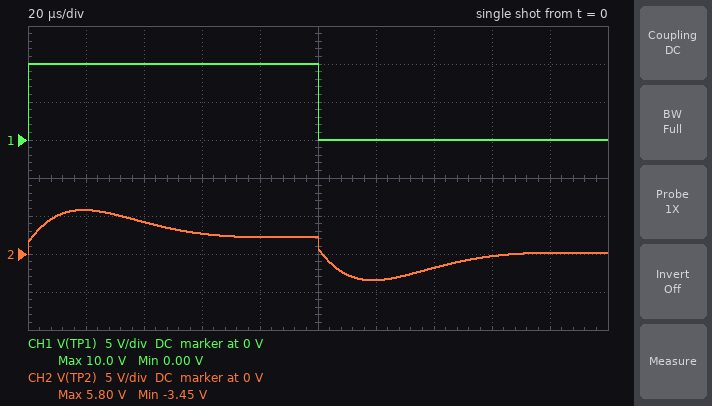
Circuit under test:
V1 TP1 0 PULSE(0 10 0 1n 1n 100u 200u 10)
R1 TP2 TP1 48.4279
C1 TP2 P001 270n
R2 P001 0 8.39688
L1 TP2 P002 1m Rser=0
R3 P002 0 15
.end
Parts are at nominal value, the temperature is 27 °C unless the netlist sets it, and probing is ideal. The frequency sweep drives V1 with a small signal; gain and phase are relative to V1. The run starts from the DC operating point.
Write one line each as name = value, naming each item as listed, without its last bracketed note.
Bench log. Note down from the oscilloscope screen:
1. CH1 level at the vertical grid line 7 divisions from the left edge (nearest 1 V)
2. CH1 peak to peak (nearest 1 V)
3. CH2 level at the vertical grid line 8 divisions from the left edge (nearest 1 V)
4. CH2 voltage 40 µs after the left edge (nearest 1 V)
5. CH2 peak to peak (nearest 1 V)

CH1 level at the vertical grid line 7 divisions from the left edge = 0 V
CH1 peak to peak = 10 V
CH2 level at the vertical grid line 8 divisions from the left edge = 0 V
CH2 voltage 40 µs after the left edge = 4 V
CH2 peak to peak = 9 V
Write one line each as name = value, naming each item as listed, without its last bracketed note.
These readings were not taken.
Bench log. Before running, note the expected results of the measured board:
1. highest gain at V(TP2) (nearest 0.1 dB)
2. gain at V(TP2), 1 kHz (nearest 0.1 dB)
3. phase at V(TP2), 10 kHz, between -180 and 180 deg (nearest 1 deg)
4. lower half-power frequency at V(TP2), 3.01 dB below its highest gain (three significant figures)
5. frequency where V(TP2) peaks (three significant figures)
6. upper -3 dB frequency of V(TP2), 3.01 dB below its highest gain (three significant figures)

highest gain at V(TP2) = -2.2 dB
gain at V(TP2), 1 kHz = -11.8 dB
phase at V(TP2), 10 kHz, between -180 and 180 deg = -3 deg
lower half-power frequency at V(TP2), 3.01 dB below its highest gain = 5.04 kHz
frequency where V(TP2) peaks = 10.1 kHz
upper -3 dB frequency of V(TP2), 3.01 dB below its highest gain = 19.5 kHz
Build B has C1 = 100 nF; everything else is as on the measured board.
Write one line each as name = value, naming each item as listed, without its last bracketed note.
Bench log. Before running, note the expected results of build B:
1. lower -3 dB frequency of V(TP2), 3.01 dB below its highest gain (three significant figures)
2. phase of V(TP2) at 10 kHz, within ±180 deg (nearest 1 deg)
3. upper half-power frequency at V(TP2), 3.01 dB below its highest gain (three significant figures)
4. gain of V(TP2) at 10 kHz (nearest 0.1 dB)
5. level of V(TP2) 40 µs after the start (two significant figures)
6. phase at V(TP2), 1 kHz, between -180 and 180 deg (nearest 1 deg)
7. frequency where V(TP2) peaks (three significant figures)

lower -3 dB frequency of V(TP2), 3.01 dB below its highest gain = 6.87 kHz
phase of V(TP2) at 10 kHz, within ±180 deg = 20 deg
upper half-power frequency at V(TP2), 3.01 dB below its highest gain = 39.3 kHz
gain of V(TP2) at 10 kHz = -2.0 dB
level of V(TP2) 40 µs after the start = 3.1 V
phase at V(TP2), 1 kHz, between -180 and 180 deg = 17 deg
frequency where V(TP2) peaks = 16.6 kHz
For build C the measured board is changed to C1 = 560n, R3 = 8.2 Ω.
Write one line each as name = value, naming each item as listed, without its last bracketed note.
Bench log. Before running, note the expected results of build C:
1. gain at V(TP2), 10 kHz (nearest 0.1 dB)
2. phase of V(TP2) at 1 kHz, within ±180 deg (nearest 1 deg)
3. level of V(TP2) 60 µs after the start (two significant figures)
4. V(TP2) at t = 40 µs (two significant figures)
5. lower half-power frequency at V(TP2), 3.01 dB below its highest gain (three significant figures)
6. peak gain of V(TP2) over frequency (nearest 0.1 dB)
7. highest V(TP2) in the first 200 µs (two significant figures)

gain at V(TP2), 10 kHz = -4.9 dB
phase of V(TP2) at 1 kHz, within ±180 deg = 30 deg
level of V(TP2) 60 µs after the start = 3.0 V
V(TP2) at t = 40 µs = 4.3 V
lower half-power frequency at V(TP2), 3.01 dB below its highest gain = 3.87 kHz
peak gain of V(TP2) over frequency = -3.1 dB
highest V(TP2) in the first 200 µs = 4.6 V
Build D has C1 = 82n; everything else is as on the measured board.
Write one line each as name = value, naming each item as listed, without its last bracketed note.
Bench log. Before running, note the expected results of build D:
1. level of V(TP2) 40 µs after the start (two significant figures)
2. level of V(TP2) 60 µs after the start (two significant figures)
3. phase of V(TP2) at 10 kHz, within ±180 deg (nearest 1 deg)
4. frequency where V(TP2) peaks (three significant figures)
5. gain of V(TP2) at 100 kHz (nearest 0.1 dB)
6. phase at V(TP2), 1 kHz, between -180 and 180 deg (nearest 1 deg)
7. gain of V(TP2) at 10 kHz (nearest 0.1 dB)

level of V(TP2) 40 µs after the start = 3.0 V
level of V(TP2) 60 µs after the start = 2.5 V
phase of V(TP2) at 10 kHz, within ±180 deg = 22 deg
frequency where V(TP2) peaks = 18.4 kHz
gain of V(TP2) at 100 kHz = -8.9 dB
phase at V(TP2), 1 kHz, between -180 and 180 deg = 17 deg
gain of V(TP2) at 10 kHz = -2.1 dB
